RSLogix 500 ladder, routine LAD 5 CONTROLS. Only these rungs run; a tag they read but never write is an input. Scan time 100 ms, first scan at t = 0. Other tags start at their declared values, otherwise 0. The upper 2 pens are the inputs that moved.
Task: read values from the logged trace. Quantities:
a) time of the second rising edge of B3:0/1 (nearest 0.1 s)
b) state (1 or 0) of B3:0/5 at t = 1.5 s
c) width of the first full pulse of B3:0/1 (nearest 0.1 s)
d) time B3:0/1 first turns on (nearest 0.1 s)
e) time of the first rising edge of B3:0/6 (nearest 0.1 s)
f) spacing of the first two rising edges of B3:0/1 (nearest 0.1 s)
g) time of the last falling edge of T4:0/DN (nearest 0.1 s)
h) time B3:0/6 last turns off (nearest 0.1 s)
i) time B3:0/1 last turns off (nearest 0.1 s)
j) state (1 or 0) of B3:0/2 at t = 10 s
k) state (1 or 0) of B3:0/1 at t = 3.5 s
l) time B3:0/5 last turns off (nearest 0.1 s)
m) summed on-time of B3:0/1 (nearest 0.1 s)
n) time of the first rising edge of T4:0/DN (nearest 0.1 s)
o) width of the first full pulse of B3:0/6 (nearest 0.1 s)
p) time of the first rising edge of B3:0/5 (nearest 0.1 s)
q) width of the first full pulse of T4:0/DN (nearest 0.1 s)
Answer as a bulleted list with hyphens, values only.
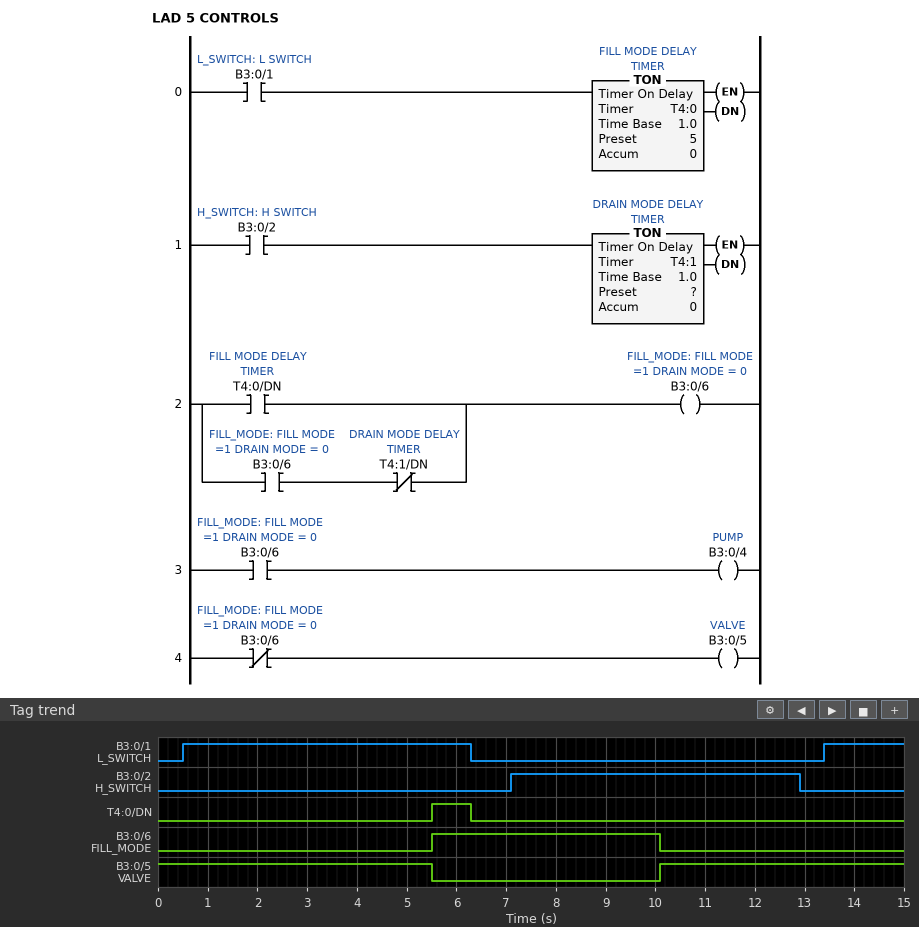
- 13.4 s
- 1
- 5.8 s
- 0.5 s
- 5.5 s
- 12.9 s
- 6.3 s
- 10.1 s
- 6.3 s
- 1
- 1
- 5.5 s
- 7.4 s
- 5.5 s
- 4.6 s
- 10.1 s
- 0.8 s
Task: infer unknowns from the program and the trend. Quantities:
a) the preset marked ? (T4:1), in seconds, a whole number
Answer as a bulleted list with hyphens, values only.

- 3 s
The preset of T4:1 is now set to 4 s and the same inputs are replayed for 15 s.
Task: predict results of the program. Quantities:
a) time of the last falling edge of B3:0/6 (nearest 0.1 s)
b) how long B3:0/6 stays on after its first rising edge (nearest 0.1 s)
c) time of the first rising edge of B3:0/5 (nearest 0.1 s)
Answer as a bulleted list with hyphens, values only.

- 11.1 s
- 5.6 s
- 11.1 s
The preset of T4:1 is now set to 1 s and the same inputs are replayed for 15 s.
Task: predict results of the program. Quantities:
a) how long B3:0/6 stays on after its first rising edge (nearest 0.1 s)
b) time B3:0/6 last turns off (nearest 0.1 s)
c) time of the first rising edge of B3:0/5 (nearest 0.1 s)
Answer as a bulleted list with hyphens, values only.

- 2.6 s
- 8.1 s
- 8.1 s
